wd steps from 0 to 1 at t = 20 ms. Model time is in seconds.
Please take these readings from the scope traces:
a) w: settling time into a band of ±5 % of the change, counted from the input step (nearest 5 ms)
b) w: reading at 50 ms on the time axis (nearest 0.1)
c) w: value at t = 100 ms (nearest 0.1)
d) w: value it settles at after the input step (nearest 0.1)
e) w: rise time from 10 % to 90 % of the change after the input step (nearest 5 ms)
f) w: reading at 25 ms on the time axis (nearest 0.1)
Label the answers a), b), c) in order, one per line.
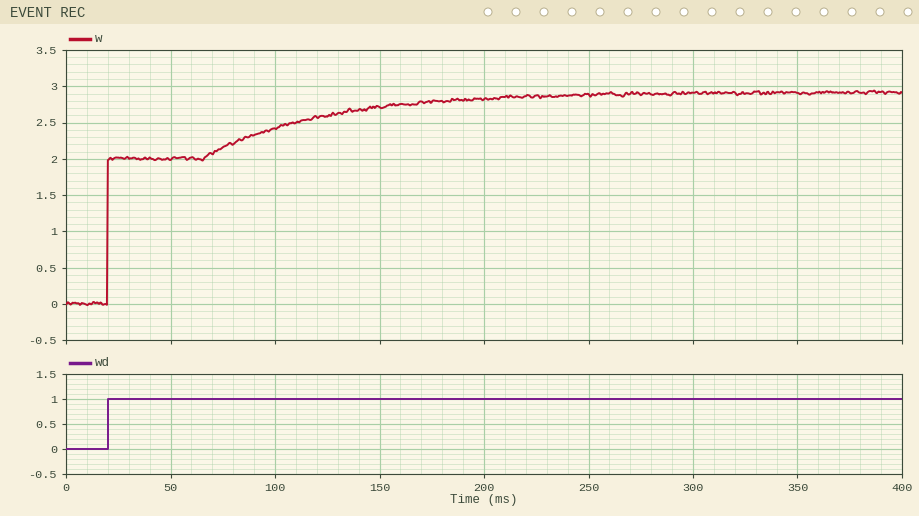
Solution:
a) 150 ms
b) 2.0
c) 2.4
d) 2.9
e) 110 ms
f) 2.0
